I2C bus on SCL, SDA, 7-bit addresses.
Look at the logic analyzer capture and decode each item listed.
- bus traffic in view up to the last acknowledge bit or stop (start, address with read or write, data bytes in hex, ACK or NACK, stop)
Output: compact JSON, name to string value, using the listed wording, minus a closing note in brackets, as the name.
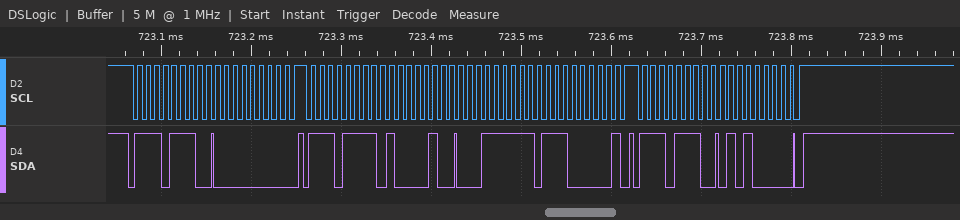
{"bus traffic in view up to the last acknowledge bit or stop": "start, address 77 write ACK, 00 ACK, stop, start, address 77 read ACK, 84 ACK, 3F ACK, E0 NACK, stop, start, address 77 write ACK, 50 ACK, stop"}
